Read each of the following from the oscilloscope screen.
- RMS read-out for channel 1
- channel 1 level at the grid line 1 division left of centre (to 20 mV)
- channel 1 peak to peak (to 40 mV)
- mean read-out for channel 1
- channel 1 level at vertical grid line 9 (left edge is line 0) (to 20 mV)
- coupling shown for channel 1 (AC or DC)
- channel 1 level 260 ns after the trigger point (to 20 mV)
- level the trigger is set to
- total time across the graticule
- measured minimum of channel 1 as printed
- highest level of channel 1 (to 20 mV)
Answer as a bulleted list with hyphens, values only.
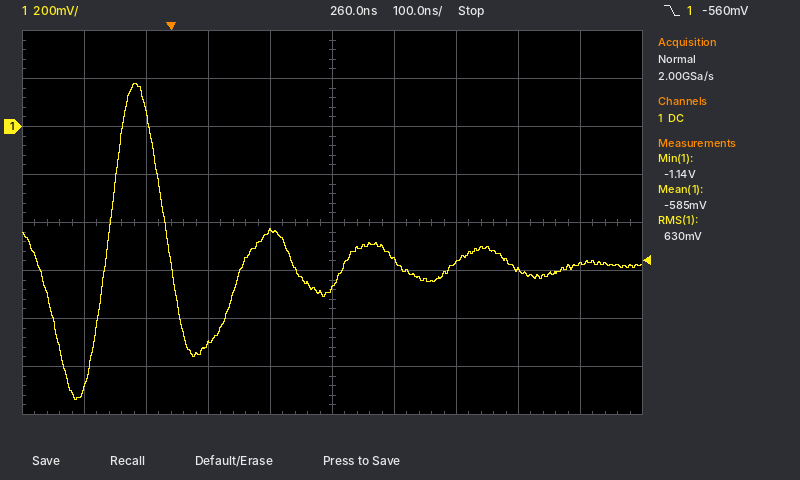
- 630 mV
- -440 mV
- 1.32 V
- -585 mV
- -580 mV
- DC
- -680 mV
- -560 mV
- 1 µs
- -1.14 V
- 180 mV
